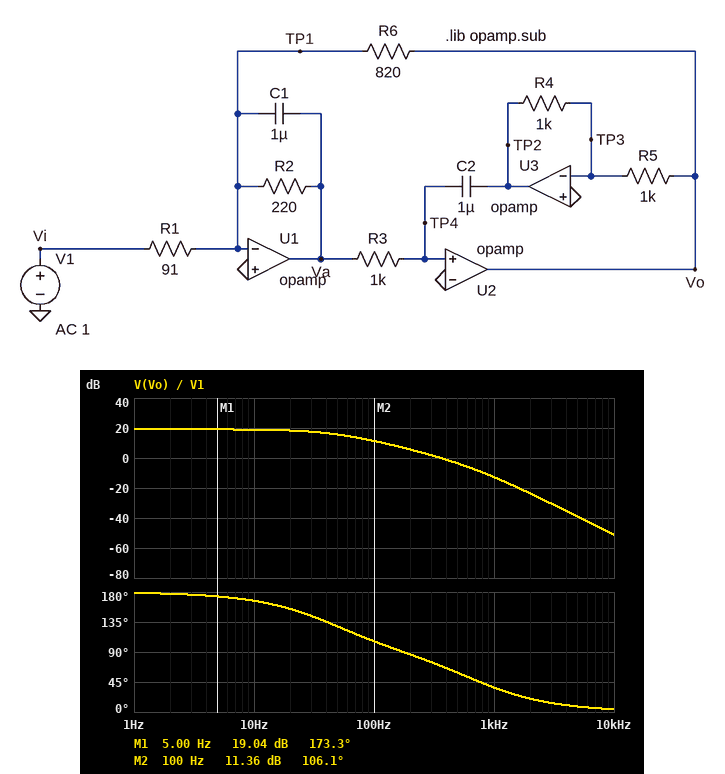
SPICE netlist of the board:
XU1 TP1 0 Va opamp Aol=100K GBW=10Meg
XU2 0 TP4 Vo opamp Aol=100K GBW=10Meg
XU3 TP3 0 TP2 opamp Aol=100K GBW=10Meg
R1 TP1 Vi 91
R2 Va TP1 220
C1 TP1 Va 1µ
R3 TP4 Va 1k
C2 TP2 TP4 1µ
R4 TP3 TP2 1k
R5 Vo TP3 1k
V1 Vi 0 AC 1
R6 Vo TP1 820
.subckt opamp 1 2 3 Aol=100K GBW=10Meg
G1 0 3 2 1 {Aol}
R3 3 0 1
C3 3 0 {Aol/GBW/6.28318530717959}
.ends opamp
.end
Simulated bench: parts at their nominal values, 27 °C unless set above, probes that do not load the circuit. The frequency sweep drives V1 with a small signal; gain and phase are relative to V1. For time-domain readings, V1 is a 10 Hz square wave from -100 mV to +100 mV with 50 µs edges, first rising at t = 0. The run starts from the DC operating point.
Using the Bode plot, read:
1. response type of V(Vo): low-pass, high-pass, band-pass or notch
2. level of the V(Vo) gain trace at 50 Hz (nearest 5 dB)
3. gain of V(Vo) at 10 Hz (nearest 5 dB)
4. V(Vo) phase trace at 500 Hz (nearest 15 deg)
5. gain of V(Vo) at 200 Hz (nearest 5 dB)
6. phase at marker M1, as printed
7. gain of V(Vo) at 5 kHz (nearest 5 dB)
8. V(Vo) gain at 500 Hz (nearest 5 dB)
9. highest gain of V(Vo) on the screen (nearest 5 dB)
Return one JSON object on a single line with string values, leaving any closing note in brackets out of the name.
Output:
{"response type of V(Vo): low-pass, high-pass, band-pass or notch": "low-pass", "level of the V(Vo) gain trace at 50 Hz": "15 dB", "gain of V(Vo) at 10 Hz": "20 dB", "V(Vo) phase trace at 500 Hz": "60 deg", "gain of V(Vo) at 200 Hz": "5 dB", "phase at marker M1, as printed": "173.3 deg", "gain of V(Vo) at 5 kHz": "-40 dB", "V(Vo) gain at 500 Hz": "-5 dB", "highest gain of V(Vo) on the screen": "20 dB"}
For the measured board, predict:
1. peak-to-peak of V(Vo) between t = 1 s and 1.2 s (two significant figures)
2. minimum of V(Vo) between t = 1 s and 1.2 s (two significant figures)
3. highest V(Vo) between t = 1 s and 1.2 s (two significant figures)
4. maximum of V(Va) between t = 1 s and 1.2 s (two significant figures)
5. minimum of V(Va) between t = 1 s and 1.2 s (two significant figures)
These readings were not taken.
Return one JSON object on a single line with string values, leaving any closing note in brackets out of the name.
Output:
{"peak-to-peak of V(Vo) between t = 1 s and 1.2 s": "1.8 V", "minimum of V(Vo) between t = 1 s and 1.2 s": "-900 mV", "highest V(Vo) between t = 1 s and 1.2 s": "900 mV", "maximum of V(Va) between t = 1 s and 1.2 s": "430 mV", "minimum of V(Va) between t = 1 s and 1.2 s": "-430 mV"}
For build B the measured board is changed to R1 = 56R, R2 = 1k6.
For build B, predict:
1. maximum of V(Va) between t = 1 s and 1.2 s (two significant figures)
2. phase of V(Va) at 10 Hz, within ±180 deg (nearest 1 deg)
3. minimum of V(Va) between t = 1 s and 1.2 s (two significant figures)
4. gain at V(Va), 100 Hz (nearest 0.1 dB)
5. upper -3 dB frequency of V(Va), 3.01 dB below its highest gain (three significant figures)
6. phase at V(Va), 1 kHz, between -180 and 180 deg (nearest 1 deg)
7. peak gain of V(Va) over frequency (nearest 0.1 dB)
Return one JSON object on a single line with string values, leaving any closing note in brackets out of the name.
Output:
{"maximum of V(Va) between t = 1 s and 1.2 s": "2.2 V", "phase of V(Va) at 10 Hz, within ±180 deg": "-92 deg", "minimum of V(Va) between t = 1 s and 1.2 s": "-2.2 V", "gain at V(Va), 100 Hz": "21.8 dB", "upper -3 dB frequency of V(Va), 3.01 dB below its highest gain": "232 Hz", "phase at V(Va), 1 kHz, between -180 and 180 deg": "96 deg", "peak gain of V(Va) over frequency": "29.1 dB"}
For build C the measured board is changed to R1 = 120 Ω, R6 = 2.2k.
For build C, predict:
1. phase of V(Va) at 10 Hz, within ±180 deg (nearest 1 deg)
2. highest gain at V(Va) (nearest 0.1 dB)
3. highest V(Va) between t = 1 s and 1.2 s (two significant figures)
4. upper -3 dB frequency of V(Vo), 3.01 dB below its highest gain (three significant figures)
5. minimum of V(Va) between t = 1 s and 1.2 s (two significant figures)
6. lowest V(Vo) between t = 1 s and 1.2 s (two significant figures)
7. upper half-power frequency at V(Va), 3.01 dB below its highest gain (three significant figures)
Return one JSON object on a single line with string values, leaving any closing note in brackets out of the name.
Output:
{"phase of V(Va) at 10 Hz, within ±180 deg": "-122 deg", "highest gain at V(Va)": "5.3 dB", "highest V(Va) between t = 1 s and 1.2 s": "340 mV", "upper -3 dB frequency of V(Vo), 3.01 dB below its highest gain": "16.3 Hz", "minimum of V(Va) between t = 1 s and 1.2 s": "-340 mV", "lowest V(Vo) between t = 1 s and 1.2 s": "-1.8 V", "upper half-power frequency at V(Va), 3.01 dB below its highest gain": "739 Hz"}
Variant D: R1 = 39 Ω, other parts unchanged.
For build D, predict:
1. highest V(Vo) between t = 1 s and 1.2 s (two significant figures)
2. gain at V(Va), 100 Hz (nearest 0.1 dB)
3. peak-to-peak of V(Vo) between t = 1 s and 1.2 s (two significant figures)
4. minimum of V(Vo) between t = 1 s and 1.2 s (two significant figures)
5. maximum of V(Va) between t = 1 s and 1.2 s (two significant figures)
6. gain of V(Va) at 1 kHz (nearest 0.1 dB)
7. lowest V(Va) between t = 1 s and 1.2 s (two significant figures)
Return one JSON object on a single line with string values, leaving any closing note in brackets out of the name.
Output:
{"highest V(Vo) between t = 1 s and 1.2 s": "2.1 V", "gain at V(Va), 100 Hz": "14.7 dB", "peak-to-peak of V(Vo) between t = 1 s and 1.2 s": "4.2 V", "minimum of V(Vo) between t = 1 s and 1.2 s": "-2.1 V", "maximum of V(Va) between t = 1 s and 1.2 s": "1.0 V", "gain of V(Va) at 1 kHz": "10.6 dB", "lowest V(Va) between t = 1 s and 1.2 s": "-1.0 V"}
